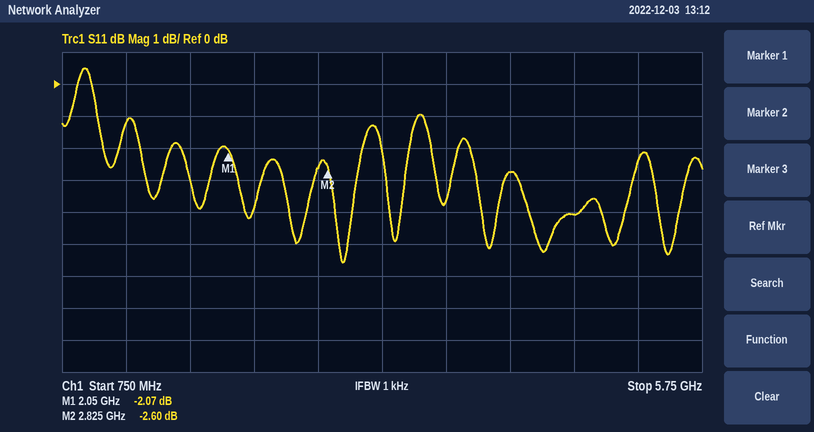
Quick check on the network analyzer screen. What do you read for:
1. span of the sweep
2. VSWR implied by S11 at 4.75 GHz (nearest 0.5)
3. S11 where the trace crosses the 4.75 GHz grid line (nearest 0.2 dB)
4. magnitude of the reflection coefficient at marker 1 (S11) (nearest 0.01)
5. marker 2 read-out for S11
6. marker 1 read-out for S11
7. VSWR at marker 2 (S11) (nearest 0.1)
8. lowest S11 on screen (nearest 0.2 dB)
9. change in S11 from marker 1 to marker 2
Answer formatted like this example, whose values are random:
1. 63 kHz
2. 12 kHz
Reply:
1. 5 GHz
2. 4.5
3. -4.0 dB
4. 0.79
5. -2.60 dB
6. -2.07 dB
7. 6.7
8. -5.6 dB
9. -0.53 dB
